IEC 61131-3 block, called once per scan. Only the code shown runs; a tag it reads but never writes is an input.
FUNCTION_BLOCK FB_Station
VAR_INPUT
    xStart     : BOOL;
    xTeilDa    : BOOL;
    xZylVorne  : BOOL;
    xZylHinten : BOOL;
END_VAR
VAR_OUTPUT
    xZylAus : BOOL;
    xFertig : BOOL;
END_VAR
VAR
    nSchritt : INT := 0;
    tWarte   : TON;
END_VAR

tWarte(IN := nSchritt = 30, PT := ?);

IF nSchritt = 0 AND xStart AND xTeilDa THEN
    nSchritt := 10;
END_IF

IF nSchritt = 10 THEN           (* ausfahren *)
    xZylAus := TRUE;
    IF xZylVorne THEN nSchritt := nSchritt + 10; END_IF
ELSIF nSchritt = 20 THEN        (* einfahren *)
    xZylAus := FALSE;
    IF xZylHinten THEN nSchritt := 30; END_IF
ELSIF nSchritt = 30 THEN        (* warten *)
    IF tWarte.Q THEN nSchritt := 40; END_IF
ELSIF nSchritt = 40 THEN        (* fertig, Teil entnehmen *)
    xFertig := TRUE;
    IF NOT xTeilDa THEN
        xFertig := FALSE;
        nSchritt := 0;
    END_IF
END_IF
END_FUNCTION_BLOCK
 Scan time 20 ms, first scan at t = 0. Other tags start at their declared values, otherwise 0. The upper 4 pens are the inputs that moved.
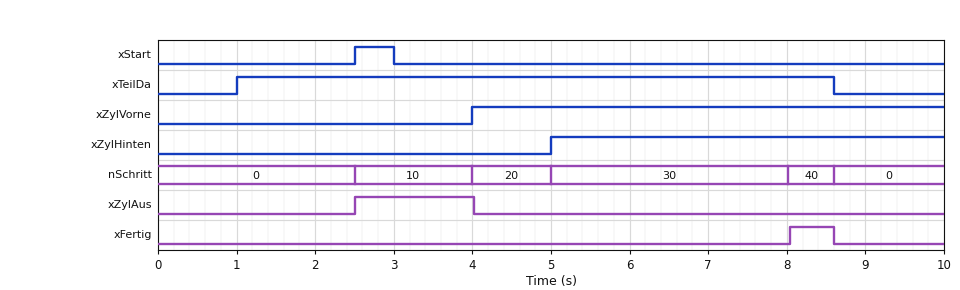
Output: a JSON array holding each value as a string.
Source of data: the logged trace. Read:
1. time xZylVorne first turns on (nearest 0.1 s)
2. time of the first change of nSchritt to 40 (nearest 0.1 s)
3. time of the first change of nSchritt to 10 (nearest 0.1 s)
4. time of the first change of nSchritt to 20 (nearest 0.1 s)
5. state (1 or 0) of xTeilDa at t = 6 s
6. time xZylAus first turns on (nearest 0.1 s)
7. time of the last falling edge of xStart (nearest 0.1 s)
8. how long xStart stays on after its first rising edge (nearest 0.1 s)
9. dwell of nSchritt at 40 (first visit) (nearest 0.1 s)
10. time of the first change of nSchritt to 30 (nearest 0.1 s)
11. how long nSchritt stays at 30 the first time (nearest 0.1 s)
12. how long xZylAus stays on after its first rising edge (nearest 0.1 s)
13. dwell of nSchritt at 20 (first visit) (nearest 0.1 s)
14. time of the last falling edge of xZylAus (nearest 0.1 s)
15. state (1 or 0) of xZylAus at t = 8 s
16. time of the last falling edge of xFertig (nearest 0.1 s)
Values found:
["4.0 s", "8.0 s", "2.5 s", "4.0 s", "1", "2.5 s", "3.0 s", "0.5 s", "0.6 s", "5.0 s", "3.0 s", "1.5 s", "1.0 s", "4.0 s", "0", "8.6 s"]
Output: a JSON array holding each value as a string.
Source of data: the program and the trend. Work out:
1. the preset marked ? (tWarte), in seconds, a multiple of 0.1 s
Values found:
["3.0 s"]
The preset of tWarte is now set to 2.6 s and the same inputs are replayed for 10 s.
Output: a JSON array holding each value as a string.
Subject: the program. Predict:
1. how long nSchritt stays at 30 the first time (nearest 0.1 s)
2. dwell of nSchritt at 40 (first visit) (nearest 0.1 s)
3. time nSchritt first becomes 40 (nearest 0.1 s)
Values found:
["2.6 s", "1.0 s", "7.6 s"]
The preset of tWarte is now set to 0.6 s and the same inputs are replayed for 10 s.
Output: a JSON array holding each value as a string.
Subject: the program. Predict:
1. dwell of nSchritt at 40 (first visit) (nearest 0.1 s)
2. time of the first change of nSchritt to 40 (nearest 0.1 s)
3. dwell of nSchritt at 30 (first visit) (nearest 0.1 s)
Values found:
["3.0 s", "5.6 s", "0.6 s"]
